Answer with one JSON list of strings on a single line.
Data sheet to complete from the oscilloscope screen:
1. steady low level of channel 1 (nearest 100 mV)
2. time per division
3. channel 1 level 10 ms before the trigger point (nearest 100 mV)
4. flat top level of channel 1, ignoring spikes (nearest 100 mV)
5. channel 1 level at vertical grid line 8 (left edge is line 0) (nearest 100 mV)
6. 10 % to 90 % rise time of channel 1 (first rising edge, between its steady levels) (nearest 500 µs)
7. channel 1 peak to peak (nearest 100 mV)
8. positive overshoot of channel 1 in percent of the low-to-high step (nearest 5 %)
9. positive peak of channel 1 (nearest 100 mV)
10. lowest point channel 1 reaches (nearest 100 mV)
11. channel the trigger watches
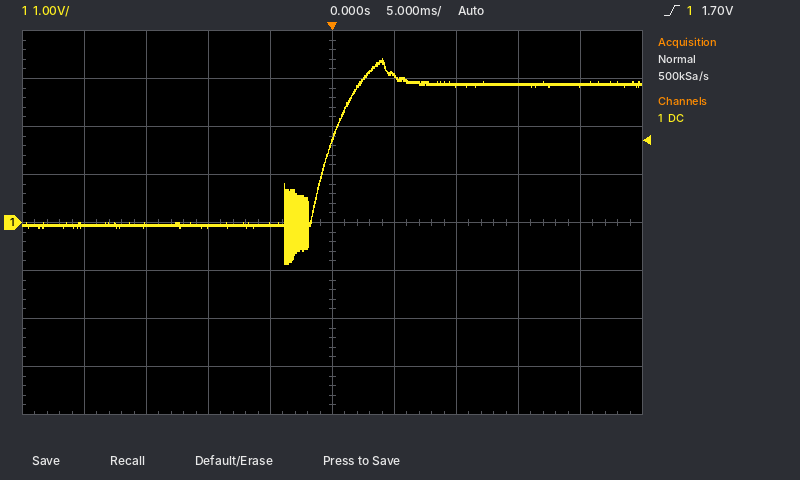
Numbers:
["-100 mV", "5 ms", "-100 mV", "2.9 V", "2.9 V", "3.0 ms", "4.3 V", "20 %", "3.4 V", "-900 mV", "channel 1"]
